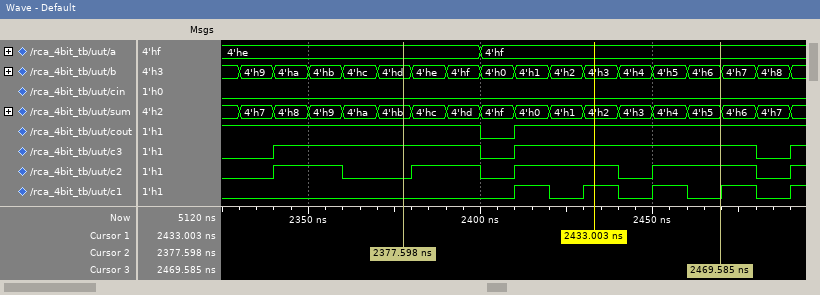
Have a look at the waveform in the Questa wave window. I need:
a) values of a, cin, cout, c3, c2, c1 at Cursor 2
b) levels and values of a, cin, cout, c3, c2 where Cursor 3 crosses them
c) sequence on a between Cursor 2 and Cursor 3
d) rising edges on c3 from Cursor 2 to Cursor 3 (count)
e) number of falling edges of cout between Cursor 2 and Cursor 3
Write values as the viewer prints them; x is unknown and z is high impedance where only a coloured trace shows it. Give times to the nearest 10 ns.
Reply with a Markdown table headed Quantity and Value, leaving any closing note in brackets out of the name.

| Quantity | Value |
|---|---|
| values of a, cin, cout, c3, c2, c1 at Cursor 2 | a=4'he, cin=0, cout=1, c3=1, c2=0, c1=0 |
| levels and values of a, cin, cout, c3, c2 where Cursor 3 crosses them | a=4'hf, cin=0, cout=1, c3=1, c2=1 |
| sequence on a between Cursor 2 and Cursor 3 | 4'he, 4'hf |
| rising edges on c3 from Cursor 2 to Cursor 3 | 1 |
| number of falling edges of cout between Cursor 2 and Cursor 3 | 1 |
